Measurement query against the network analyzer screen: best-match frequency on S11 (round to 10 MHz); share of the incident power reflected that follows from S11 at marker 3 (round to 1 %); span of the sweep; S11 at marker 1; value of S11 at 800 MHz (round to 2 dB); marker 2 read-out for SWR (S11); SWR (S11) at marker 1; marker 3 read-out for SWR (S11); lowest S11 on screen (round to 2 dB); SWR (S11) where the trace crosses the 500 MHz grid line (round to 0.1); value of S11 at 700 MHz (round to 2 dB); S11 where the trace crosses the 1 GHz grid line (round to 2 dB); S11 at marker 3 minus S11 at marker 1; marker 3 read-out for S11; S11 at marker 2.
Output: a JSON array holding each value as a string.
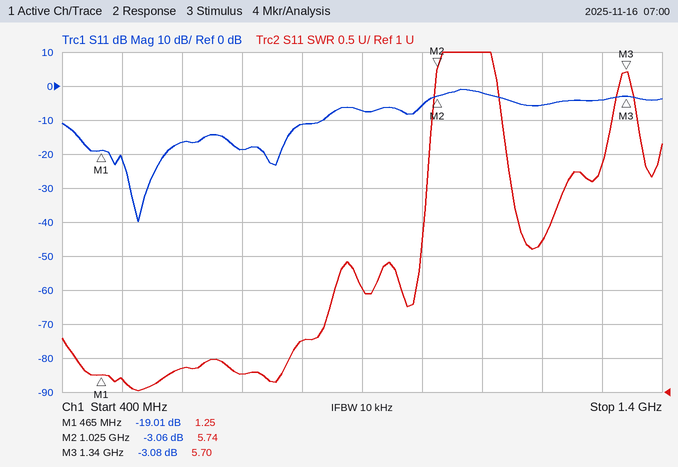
["530 MHz", "49 %", "1 GHz", "-19.01 dB", "-12 dB", "5.74", "1.25", "5.70", "-40 dB", "1.2", "-18 dB", "-6 dB", "15.93 dB", "-3.08 dB", "-3.06 dB"]
